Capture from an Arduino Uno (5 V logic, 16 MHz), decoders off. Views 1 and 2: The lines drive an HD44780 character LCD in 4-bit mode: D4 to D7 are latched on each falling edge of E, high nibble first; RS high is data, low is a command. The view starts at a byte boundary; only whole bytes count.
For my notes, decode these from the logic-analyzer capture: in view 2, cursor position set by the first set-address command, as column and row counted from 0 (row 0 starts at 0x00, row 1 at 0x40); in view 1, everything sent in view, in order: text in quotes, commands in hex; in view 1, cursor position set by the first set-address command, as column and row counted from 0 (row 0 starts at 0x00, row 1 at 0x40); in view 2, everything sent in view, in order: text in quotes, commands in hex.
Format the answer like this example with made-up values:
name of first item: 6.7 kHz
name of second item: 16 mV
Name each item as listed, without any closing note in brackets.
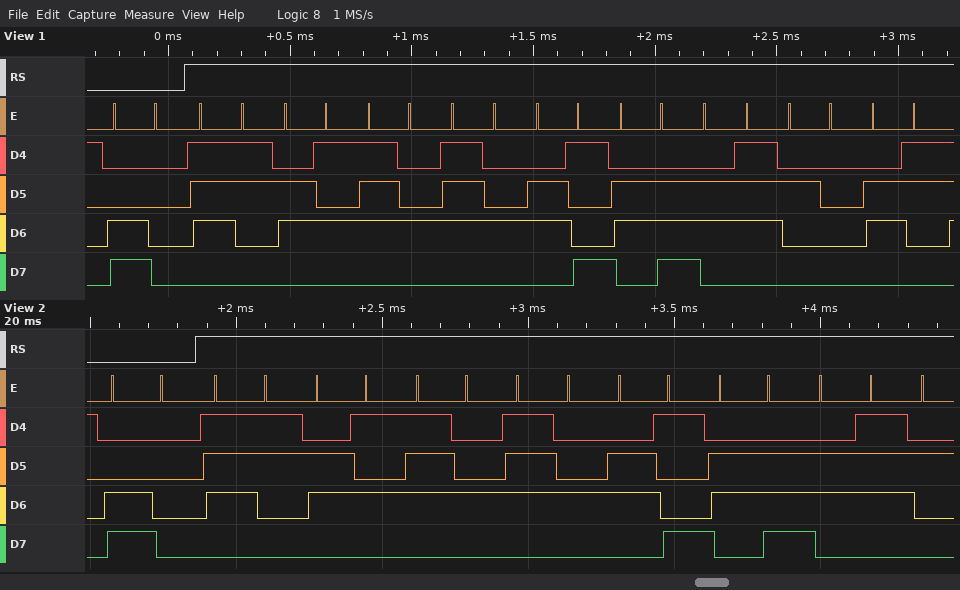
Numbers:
in view 2, cursor position set by the first set-address command, as column and row counted from 0: column 0, row 1
in view 1, everything sent in view, in order: text in quotes, commands in hex: 0xC0 "setting c"
in view 1, cursor position set by the first set-address command, as column and row counted from 0: column 0, row 1
in view 2, everything sent in view, in order: text in quotes, commands in hex: 0xC0 "setting"
